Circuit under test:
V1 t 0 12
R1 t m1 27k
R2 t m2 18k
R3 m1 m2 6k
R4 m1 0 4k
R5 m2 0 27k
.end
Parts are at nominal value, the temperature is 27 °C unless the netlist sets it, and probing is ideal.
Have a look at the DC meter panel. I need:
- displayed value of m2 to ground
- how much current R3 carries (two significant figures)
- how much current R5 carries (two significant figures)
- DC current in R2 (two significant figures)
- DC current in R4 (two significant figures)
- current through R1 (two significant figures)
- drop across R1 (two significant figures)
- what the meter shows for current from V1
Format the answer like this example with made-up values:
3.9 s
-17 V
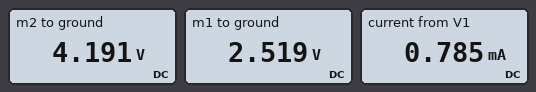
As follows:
4.191 V
280 µA
160 µA
430 µA
630 µA
350 µA
9.5 V
0.785 mA
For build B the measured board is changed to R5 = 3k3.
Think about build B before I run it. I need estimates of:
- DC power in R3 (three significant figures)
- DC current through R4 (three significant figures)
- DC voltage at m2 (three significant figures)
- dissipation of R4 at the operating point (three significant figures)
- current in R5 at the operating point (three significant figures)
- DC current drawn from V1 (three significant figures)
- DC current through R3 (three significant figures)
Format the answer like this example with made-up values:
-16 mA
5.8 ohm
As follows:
3.85 µW
409 µA
1.79 V
670 µW
542 µA
951 µA
25.3 µA
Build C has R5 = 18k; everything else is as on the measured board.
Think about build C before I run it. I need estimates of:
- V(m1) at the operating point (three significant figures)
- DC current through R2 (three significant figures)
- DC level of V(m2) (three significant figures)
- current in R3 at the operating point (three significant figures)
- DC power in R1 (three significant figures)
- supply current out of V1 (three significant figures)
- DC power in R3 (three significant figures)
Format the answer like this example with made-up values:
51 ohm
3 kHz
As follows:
2.39 V
454 µA
3.83 V
241 µA
3.42 mW
810 µA
348 µW
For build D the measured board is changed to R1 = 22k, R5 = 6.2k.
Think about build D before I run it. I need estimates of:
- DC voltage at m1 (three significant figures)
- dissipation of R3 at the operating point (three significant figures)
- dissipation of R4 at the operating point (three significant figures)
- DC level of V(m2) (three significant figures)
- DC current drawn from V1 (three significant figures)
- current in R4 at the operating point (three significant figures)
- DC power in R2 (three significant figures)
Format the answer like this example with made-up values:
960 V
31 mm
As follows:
2.14 V
46.2 µW
1.15 mW
2.67 V
966 µA
536 µA
4.84 mW
